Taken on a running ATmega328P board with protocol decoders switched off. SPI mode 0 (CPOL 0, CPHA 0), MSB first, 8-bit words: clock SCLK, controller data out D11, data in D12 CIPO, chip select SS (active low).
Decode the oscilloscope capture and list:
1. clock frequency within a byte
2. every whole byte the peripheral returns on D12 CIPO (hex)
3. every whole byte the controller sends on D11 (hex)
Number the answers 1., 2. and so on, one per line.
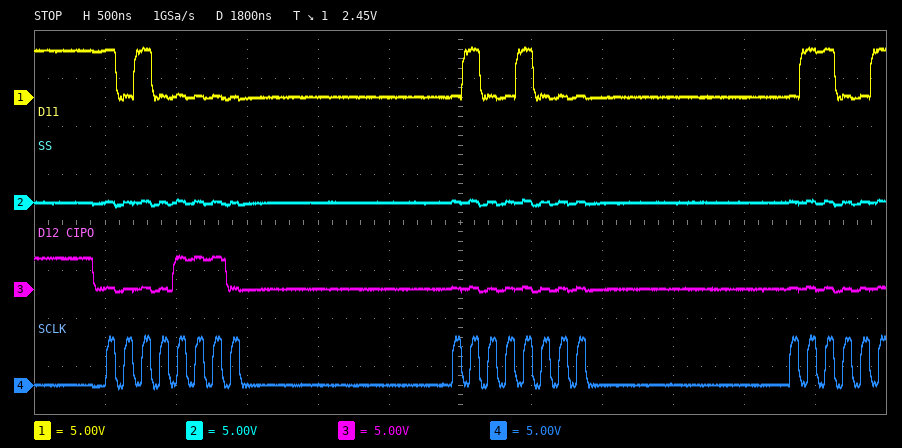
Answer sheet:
1. 8 MHz
2. 0E 00
3. A0 48
